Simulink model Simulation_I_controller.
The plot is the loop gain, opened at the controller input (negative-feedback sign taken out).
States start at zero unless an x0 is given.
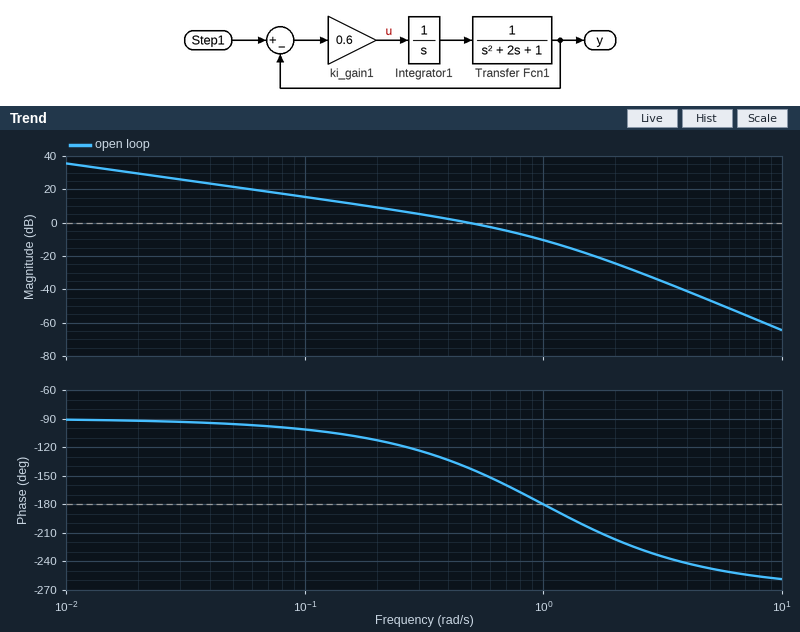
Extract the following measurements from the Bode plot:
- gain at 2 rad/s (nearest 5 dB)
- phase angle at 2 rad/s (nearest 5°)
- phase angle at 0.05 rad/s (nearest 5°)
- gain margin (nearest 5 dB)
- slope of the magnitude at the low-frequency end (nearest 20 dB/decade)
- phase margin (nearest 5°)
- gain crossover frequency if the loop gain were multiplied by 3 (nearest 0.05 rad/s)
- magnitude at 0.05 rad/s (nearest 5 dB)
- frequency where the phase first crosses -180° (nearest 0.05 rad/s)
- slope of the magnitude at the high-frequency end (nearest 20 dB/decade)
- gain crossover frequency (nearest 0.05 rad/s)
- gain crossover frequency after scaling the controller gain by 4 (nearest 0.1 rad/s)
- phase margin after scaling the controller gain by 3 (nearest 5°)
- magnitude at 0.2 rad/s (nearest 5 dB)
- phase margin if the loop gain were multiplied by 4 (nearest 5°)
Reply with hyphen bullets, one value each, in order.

- -25 dB
- -215°
- -95°
- 10 dB
- -20 dB/decade
- 40°
- 0.95 rad/s
- 20 dB
- 1.00 rad/s
- -60 dB/decade
- 0.50 rad/s
- 1.1 rad/s
- 5°
- 10 dB
- -5°
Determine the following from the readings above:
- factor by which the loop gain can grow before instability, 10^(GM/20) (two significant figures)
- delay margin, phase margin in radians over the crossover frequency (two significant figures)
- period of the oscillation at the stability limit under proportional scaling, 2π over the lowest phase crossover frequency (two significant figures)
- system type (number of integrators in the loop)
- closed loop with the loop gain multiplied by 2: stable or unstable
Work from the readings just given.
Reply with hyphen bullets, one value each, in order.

- 3.2
- 1.4 s
- 6.3 s
- 1
- stable
